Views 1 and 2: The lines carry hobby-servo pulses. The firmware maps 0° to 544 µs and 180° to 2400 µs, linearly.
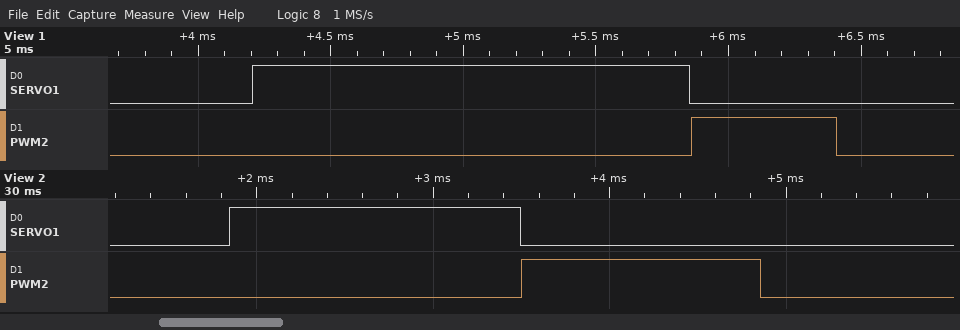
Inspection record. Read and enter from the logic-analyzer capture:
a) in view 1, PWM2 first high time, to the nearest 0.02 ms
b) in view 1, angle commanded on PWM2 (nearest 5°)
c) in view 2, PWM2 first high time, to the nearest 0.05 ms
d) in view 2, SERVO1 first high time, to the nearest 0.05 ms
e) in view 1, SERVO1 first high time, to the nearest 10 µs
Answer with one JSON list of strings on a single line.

["0.54 ms", "0°", "1.35 ms", "1.65 ms", "1650 µs"]
